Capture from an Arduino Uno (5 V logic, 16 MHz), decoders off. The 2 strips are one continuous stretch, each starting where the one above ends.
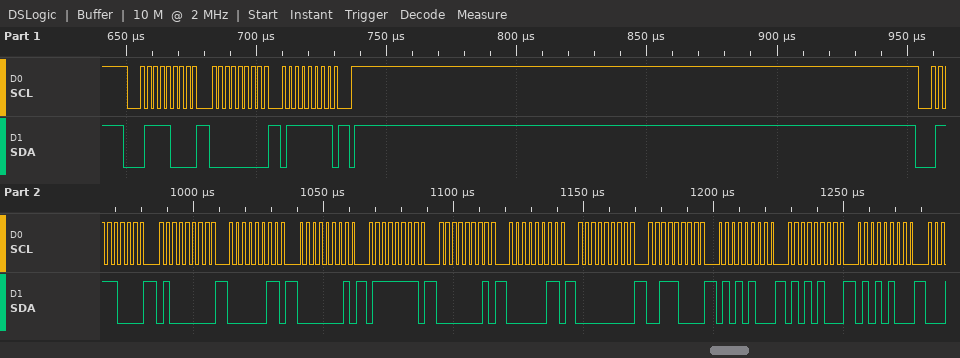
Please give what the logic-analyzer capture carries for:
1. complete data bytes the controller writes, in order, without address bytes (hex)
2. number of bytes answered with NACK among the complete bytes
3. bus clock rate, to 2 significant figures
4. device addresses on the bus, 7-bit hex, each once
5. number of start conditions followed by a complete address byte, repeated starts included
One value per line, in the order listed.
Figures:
00 7F 40 03 01 7F 01 03 00 38 54 54 54
0
400 kHz
0x3C
2
